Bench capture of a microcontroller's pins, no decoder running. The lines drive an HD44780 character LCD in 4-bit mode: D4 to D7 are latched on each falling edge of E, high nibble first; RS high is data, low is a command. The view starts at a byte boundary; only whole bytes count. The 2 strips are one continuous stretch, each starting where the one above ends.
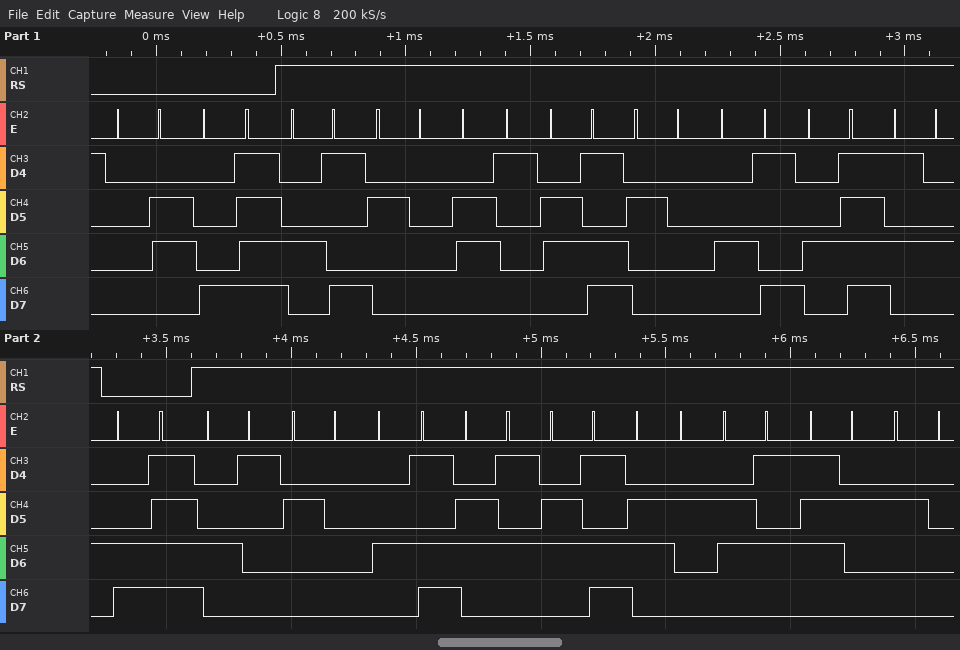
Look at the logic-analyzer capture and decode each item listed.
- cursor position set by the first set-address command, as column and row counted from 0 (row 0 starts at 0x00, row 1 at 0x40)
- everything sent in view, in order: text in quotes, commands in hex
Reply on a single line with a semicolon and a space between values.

column 15, row 0; 0x06 0x8F "I am IOT" 0xCF "A Member "
